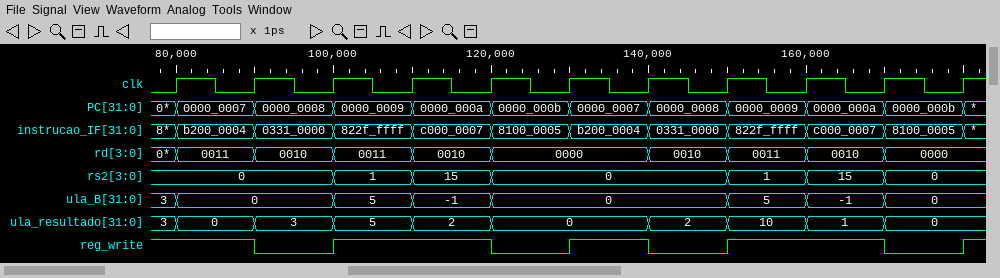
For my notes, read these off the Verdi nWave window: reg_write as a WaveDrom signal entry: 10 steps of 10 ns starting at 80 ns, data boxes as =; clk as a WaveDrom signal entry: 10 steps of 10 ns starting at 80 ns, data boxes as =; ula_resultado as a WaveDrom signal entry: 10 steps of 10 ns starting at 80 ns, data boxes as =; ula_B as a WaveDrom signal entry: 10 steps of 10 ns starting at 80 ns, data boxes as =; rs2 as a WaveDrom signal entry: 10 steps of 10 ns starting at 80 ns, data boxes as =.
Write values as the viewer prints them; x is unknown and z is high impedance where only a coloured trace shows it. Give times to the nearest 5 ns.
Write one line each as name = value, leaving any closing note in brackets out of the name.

reg_write as a WaveDrom signal entry: 10 steps of 10 ns starting at 80 ns, data boxes as = = {name: 'reg_write', wave: '101.0101.0'}
clk as a WaveDrom signal entry: 10 steps of 10 ns starting at 80 ns, data boxes as = = {name: 'clk', wave: 'p.........'}
ula_resultado as a WaveDrom signal entry: 10 steps of 10 ns starting at 80 ns, data boxes as = = {name: 'ula_resultado', wave: '=====.====', data: '0 3 5 2 0 2 10 1 0'}
ula_B as a WaveDrom signal entry: 10 steps of 10 ns starting at 80 ns, data boxes as = = {name: 'ula_B', wave: '=.===..===', data: '0 5 -1 0 5 -1 0'}
rs2 as a WaveDrom signal entry: 10 steps of 10 ns starting at 80 ns, data boxes as = = {name: 'rs2', wave: '=.===..===', data: '0 1 15 0 1 15 0'}
